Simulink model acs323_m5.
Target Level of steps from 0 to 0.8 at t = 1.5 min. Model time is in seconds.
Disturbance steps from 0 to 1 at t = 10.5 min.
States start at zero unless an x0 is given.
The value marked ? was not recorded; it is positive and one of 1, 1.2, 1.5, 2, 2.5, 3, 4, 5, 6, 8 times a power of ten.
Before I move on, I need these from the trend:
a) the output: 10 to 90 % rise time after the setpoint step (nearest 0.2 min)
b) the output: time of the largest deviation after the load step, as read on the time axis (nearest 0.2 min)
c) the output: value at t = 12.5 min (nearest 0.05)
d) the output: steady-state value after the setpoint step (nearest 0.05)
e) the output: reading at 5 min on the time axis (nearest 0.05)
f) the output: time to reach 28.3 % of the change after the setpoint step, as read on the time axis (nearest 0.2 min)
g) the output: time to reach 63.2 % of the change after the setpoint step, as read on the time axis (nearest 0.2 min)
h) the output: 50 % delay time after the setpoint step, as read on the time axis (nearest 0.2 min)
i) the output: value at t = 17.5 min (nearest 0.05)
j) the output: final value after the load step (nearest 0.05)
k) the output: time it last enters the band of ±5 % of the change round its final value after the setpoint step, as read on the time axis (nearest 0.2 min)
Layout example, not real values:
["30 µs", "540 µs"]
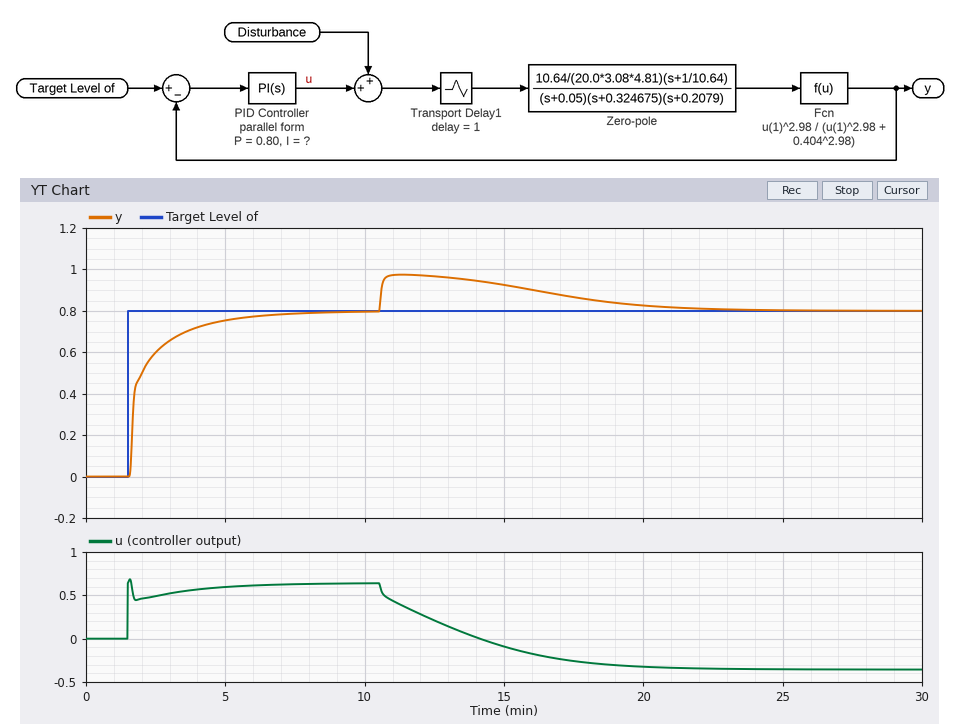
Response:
["2.4 min", "11.4 min", "0.95", "0.80", "0.75", "1.6 min", "2.0 min", "1.8 min", "0.85", "0.80", "5.2 min"]
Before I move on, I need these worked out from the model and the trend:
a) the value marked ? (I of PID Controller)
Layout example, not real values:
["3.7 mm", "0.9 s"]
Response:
["0.015"]
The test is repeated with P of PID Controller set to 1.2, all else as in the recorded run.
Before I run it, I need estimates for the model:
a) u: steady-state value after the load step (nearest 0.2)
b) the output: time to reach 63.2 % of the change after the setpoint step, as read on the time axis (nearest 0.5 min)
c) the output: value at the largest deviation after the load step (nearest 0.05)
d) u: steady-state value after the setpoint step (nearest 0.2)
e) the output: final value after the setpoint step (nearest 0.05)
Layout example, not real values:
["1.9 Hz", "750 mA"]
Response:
["-0.4", "1.5 min", "0.95", "0.6", "0.80"]
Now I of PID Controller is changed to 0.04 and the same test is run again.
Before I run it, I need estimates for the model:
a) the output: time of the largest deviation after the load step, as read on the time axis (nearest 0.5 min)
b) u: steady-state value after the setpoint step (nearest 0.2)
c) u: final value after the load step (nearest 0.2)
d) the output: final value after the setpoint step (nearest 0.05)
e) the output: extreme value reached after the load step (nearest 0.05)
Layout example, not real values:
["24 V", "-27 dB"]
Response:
["11.0 min", "0.6", "-0.4", "0.80", "0.95"]
